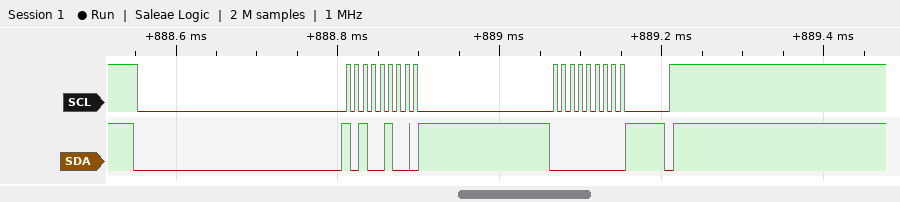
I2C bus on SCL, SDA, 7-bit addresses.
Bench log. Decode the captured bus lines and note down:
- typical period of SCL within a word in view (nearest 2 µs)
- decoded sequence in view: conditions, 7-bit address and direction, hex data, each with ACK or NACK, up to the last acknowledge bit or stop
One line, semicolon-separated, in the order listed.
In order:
10 µs; start, address 52 write ACK, 00 ACK, stop
